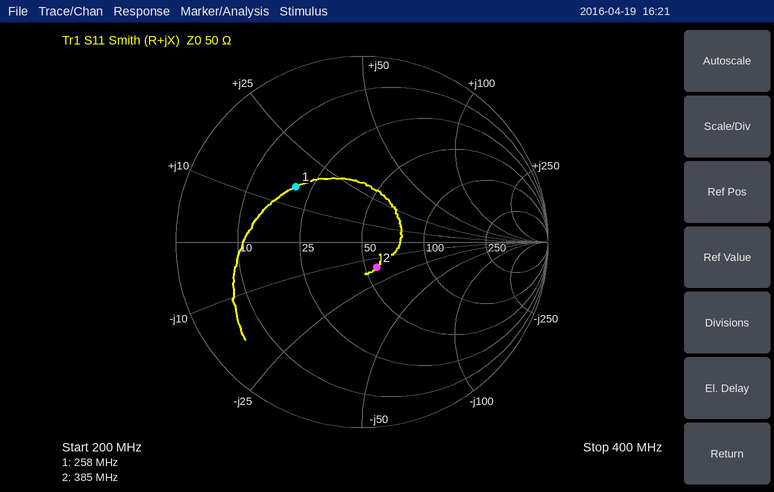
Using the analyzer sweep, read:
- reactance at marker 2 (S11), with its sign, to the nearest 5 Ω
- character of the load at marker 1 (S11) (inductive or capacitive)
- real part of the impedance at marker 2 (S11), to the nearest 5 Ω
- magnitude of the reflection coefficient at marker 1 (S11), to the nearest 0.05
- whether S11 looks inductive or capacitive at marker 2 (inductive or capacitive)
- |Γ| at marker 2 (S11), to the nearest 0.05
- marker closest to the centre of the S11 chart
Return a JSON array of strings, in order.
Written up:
["-15 Ω", "inductive", "55 Ω", "0.45", "capacitive", "0.15", "marker 2"]
